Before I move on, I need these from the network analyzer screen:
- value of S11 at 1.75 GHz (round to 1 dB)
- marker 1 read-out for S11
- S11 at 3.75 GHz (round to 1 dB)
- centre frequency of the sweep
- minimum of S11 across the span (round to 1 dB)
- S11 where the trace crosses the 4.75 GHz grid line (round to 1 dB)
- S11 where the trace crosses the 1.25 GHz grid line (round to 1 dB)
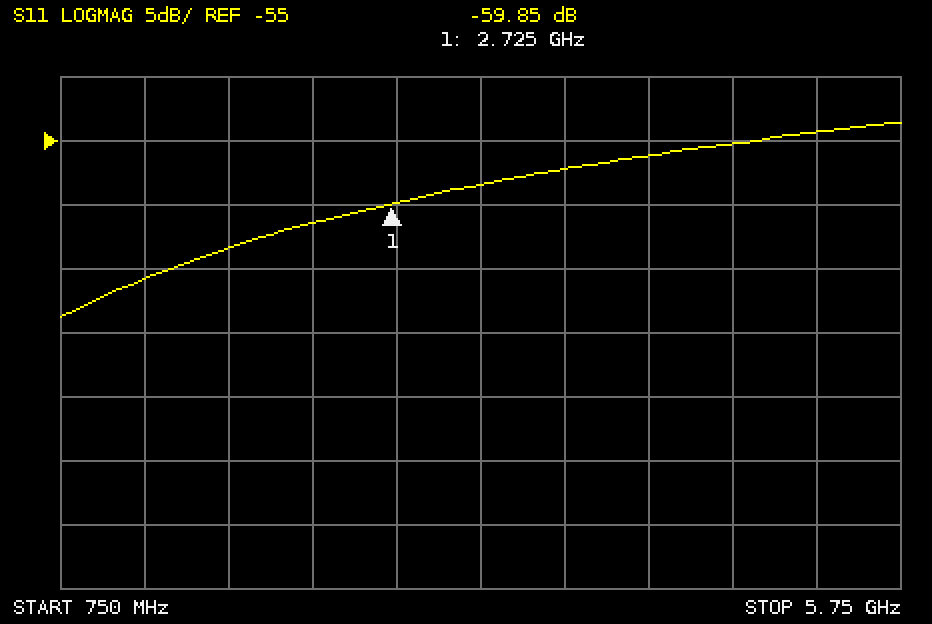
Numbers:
-63 dB
-59.85 dB
-57 dB
3.25 GHz
-69 dB
-55 dB
-66 dB
